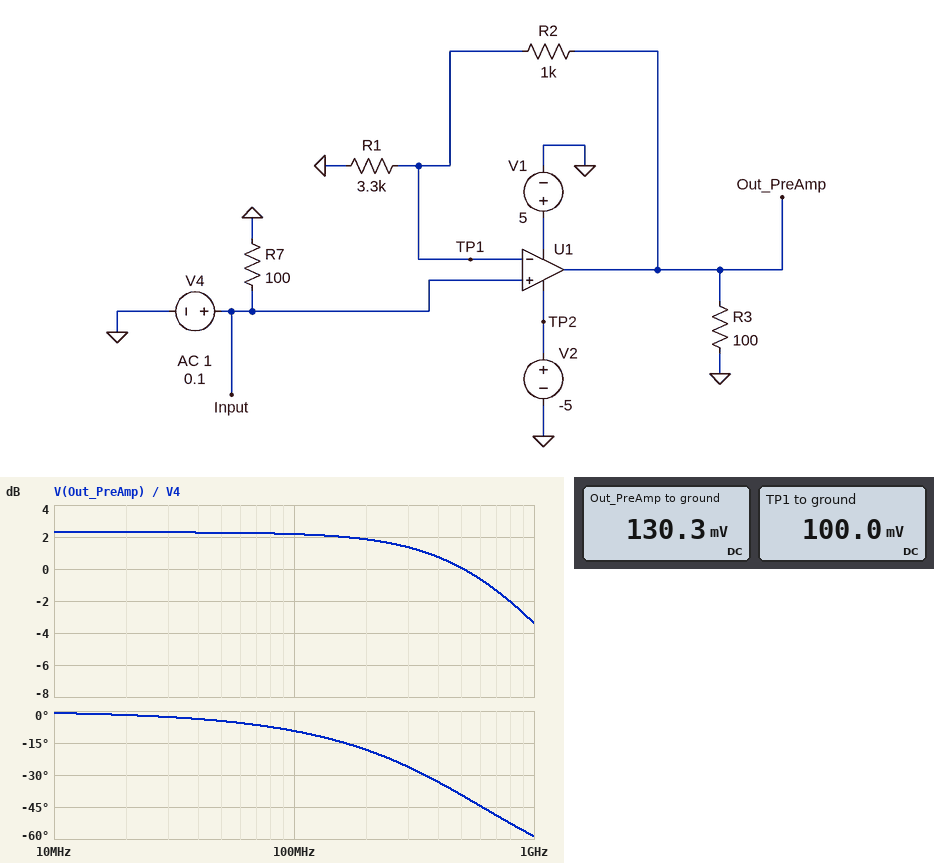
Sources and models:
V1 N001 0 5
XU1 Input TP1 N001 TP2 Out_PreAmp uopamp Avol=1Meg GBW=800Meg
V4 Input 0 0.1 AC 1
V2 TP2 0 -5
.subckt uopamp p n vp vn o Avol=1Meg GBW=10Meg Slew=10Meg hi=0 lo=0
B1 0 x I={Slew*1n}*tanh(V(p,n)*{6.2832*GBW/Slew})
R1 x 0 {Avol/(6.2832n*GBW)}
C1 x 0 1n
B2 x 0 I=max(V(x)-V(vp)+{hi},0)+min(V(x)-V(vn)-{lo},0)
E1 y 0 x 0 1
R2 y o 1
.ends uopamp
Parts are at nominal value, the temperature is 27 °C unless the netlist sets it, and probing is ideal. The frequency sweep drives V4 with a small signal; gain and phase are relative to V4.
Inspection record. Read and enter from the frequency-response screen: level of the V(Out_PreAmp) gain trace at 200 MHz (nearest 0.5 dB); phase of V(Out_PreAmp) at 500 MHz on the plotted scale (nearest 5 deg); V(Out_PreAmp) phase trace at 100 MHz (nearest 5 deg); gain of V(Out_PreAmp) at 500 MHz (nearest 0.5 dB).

2.0 dB
-40 deg
-10 deg
0 dB
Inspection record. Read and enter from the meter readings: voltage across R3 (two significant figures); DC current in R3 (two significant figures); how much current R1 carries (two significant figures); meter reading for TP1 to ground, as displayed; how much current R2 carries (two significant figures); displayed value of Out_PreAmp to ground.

130 mV
1.3 mA
30 µA
100.0 mV
30 µA
130.3 mV
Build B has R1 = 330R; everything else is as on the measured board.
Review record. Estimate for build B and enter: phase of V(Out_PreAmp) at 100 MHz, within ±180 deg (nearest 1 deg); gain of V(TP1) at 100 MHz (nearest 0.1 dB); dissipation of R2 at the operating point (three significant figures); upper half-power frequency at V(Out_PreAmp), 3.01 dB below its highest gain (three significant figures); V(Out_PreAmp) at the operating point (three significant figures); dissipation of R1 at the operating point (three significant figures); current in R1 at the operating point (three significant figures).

-27 deg
-1.0 dB
91.8 µW
196 MHz
403 mV
30.3 µW
303 µA
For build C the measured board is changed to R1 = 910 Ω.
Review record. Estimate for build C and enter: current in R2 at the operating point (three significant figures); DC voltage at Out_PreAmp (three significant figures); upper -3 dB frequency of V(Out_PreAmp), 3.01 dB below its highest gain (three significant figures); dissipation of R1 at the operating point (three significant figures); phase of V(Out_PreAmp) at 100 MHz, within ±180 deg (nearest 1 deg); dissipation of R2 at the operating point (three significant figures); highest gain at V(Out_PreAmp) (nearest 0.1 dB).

110 µA
210 mV
377 MHz
11.0 µW
-15 deg
12.1 µW
6.4 dB
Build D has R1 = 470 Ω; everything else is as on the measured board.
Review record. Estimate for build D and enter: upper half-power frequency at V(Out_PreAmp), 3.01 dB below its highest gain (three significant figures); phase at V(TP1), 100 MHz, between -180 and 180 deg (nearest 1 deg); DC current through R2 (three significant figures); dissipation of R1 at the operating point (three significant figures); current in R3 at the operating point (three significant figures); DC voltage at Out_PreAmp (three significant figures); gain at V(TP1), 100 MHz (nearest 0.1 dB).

253 MHz
-22 deg
213 µA
21.3 µW
3.13 mA
313 mV
-0.6 dB
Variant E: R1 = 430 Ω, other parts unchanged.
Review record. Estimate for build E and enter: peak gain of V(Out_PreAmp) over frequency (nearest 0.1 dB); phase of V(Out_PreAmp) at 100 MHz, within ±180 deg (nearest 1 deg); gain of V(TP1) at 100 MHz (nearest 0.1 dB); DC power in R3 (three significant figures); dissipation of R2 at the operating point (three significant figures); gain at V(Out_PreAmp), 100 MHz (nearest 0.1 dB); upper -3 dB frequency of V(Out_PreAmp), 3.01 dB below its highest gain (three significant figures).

10.4 dB
-23 deg
-0.7 dB
1.11 mW
54.1 µW
9.7 dB
238 MHz
